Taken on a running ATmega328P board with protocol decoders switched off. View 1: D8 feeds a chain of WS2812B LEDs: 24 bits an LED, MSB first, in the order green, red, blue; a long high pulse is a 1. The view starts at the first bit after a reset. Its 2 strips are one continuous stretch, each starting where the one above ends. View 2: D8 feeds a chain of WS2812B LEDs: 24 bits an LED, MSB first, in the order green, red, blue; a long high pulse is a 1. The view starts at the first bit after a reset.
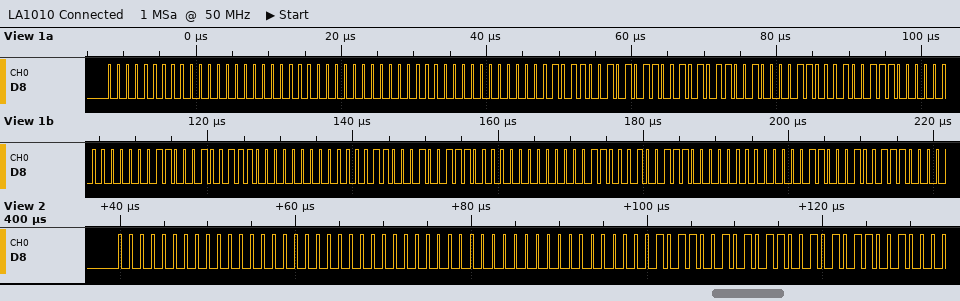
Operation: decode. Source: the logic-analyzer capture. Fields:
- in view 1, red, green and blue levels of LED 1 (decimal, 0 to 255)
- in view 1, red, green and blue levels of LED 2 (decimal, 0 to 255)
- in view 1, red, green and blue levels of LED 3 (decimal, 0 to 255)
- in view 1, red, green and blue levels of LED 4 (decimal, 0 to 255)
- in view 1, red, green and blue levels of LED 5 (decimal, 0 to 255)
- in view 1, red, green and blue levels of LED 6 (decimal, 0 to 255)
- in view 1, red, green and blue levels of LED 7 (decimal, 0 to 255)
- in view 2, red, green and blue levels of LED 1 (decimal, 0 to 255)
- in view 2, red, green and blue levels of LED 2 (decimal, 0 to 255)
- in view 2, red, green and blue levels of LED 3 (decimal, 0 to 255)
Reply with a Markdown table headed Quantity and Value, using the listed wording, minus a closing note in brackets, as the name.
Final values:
| Quantity | Value |
|---|---|
| in view 1, red, green and blue levels of LED 1 | 0, 0, 0 |
| in view 1, red, green and blue levels of LED 2 | 0, 0, 0 |
| in view 1, red, green and blue levels of LED 3 | 89, 89, 89 |
| in view 1, red, green and blue levels of LED 4 | 78, 12, 0 |
| in view 1, red, green and blue levels of LED 5 | 78, 12, 0 |
| in view 1, red, green and blue levels of LED 6 | 78, 12, 0 |
| in view 1, red, green and blue levels of LED 7 | 78, 12, 0 |
| in view 2, red, green and blue levels of LED 1 | 0, 0, 0 |
| in view 2, red, green and blue levels of LED 2 | 0, 0, 0 |
| in view 2, red, green and blue levels of LED 3 | 89, 89, 89 |
